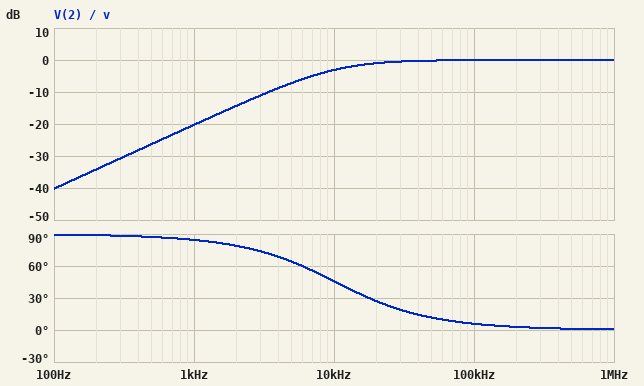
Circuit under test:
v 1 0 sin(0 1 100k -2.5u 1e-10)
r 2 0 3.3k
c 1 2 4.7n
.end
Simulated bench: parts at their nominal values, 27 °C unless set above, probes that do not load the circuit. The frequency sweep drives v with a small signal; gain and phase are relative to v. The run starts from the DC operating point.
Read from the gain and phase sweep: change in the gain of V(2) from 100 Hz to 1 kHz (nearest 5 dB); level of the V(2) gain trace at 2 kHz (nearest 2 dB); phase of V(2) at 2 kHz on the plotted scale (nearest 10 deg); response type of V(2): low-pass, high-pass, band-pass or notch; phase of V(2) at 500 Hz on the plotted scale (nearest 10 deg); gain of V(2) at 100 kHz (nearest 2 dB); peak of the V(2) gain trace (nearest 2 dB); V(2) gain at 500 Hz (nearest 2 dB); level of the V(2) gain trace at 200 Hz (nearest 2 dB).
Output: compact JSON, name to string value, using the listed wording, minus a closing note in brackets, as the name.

{"change in the gain of V(2) from 100 Hz to 1 kHz": "20 dB", "level of the V(2) gain trace at 2 kHz": "-14 dB", "phase of V(2) at 2 kHz on the plotted scale": "80 deg", "response type of V(2): low-pass, high-pass, band-pass or notch": "high-pass", "phase of V(2) at 500 Hz on the plotted scale": "90 deg", "gain of V(2) at 100 kHz": "0 dB", "peak of the V(2) gain trace": "0 dB", "V(2) gain at 500 Hz": "-26 dB", "level of the V(2) gain trace at 200 Hz": "-34 dB"}
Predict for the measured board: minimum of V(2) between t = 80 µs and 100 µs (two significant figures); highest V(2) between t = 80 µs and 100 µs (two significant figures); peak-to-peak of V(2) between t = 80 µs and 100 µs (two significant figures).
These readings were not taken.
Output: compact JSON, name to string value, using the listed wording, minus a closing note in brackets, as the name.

{"minimum of V(2) between t = 80 µs and 100 µs": "-1.0 V", "highest V(2) between t = 80 µs and 100 µs": "990 mV", "peak-to-peak of V(2) between t = 80 µs and 100 µs": "2.0 V"}
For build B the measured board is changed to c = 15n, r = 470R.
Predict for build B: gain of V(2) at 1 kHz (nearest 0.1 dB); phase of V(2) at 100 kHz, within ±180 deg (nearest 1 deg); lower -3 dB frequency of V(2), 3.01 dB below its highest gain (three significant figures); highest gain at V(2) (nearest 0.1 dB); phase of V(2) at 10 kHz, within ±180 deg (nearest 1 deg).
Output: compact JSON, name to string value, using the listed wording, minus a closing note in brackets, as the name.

{"gain of V(2) at 1 kHz": "-27.1 dB", "phase of V(2) at 100 kHz, within ±180 deg": "13 deg", "lower -3 dB frequency of V(2), 3.01 dB below its highest gain": "22.6 kHz", "highest gain at V(2)": "0 dB", "phase of V(2) at 10 kHz, within ±180 deg": "66 deg"}
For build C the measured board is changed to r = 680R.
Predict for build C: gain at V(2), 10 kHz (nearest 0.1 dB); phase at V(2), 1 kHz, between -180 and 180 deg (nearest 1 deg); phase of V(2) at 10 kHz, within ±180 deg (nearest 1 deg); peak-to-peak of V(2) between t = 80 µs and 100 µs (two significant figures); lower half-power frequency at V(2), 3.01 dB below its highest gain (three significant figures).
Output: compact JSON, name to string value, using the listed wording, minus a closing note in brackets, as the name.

{"gain at V(2), 10 kHz": "-14.1 dB", "phase at V(2), 1 kHz, between -180 and 180 deg": "89 deg", "phase of V(2) at 10 kHz, within ±180 deg": "79 deg", "peak-to-peak of V(2) between t = 80 µs and 100 µs": "1.8 V", "lower half-power frequency at V(2), 3.01 dB below its highest gain": "49.8 kHz"}
